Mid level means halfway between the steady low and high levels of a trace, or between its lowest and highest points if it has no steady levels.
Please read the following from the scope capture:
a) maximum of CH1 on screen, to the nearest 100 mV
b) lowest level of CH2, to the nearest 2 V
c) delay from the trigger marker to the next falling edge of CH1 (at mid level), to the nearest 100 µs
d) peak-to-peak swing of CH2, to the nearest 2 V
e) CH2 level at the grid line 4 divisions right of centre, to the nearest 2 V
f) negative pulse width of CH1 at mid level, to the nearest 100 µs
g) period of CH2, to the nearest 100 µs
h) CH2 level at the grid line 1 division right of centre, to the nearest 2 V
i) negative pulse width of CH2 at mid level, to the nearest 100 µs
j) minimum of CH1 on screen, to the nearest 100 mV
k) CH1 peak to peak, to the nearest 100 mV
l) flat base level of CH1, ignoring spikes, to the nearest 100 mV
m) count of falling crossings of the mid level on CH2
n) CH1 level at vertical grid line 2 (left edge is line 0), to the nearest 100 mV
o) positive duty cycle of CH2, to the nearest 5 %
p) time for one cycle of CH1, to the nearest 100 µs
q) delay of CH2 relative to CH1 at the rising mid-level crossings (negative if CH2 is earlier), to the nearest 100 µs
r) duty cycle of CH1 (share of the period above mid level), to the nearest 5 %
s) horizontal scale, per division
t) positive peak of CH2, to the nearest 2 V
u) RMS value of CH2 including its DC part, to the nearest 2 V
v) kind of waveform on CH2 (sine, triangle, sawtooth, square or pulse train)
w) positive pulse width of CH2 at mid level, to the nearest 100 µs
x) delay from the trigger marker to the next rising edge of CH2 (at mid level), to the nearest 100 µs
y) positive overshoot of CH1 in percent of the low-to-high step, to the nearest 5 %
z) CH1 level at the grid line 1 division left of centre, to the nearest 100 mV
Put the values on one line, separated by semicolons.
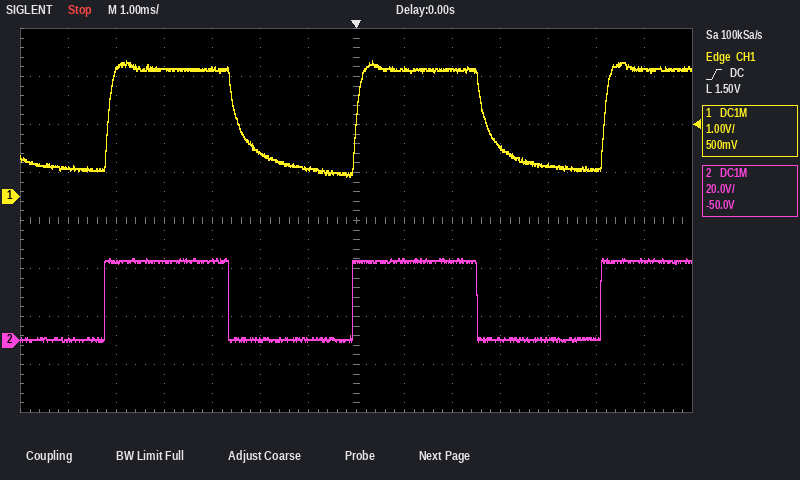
2.8 V; 0 V; 2.7 ms; 34 V; 0 V; 2.5 ms; 5.2 ms; 34 V; 2.6 ms; 400 mV; 2.4 V; 600 mV; 2; 2.6 V; 50 %; 5.2 ms; -100 µs; 50 %; 1 ms; 34 V; 24 V; square; 2.6 ms; 5.1 ms; 10 %; 600 mV
